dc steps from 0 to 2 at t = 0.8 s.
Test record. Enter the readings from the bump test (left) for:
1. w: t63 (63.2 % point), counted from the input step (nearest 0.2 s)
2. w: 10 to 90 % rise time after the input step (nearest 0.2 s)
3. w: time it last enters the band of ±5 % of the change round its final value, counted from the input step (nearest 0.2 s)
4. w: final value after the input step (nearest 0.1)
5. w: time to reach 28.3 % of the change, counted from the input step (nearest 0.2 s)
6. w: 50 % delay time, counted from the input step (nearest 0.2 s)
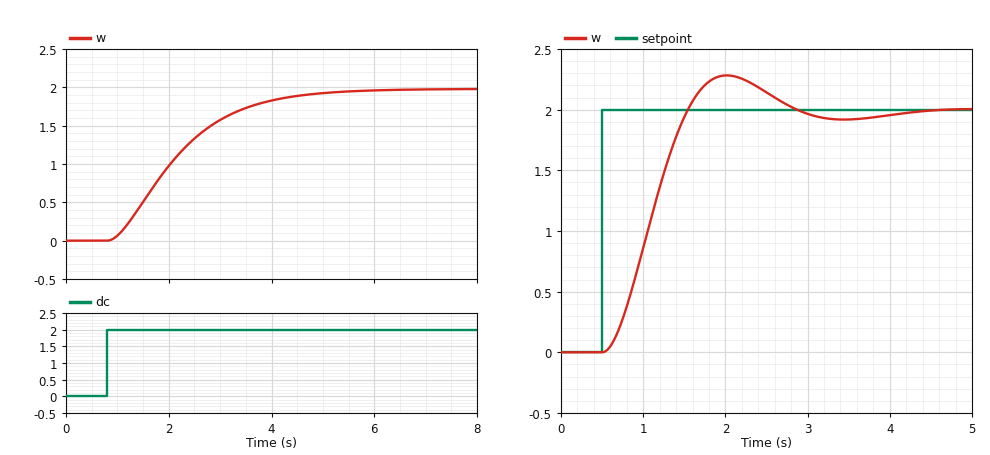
1.6 s
2.6 s
3.6 s
2.0
0.8 s
1.2 s
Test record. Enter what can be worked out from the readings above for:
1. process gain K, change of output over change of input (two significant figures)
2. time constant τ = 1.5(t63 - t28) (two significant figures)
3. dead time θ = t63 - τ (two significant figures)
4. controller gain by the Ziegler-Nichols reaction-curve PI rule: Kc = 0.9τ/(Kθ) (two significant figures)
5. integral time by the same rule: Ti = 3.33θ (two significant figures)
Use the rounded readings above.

1.0
1.2 s
0.40 s
2.7
1.3 s
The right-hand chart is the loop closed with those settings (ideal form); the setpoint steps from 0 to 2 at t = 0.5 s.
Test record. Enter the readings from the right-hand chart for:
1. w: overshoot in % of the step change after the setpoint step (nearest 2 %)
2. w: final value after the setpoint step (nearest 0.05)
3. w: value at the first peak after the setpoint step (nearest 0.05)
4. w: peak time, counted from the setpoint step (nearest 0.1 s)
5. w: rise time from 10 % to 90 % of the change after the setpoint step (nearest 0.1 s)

14 %
2.00
2.30
1.5 s
0.7 s
